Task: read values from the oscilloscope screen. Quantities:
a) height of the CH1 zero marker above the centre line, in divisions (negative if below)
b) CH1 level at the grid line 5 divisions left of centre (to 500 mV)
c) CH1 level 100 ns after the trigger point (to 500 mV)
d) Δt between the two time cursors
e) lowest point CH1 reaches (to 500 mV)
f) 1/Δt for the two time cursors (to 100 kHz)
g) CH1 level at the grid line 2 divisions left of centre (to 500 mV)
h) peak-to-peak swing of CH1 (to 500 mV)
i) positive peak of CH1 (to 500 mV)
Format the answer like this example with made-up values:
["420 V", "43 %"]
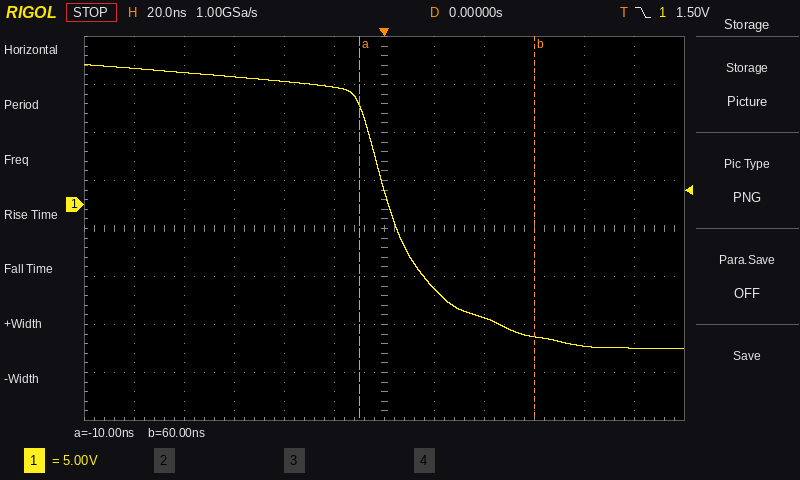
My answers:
["+0.5 div", "14.0 V", "-15.0 V", "70 ns", "-15.0 V", "14.3 MHz", "13.0 V", "29.5 V", "14.5 V"]
